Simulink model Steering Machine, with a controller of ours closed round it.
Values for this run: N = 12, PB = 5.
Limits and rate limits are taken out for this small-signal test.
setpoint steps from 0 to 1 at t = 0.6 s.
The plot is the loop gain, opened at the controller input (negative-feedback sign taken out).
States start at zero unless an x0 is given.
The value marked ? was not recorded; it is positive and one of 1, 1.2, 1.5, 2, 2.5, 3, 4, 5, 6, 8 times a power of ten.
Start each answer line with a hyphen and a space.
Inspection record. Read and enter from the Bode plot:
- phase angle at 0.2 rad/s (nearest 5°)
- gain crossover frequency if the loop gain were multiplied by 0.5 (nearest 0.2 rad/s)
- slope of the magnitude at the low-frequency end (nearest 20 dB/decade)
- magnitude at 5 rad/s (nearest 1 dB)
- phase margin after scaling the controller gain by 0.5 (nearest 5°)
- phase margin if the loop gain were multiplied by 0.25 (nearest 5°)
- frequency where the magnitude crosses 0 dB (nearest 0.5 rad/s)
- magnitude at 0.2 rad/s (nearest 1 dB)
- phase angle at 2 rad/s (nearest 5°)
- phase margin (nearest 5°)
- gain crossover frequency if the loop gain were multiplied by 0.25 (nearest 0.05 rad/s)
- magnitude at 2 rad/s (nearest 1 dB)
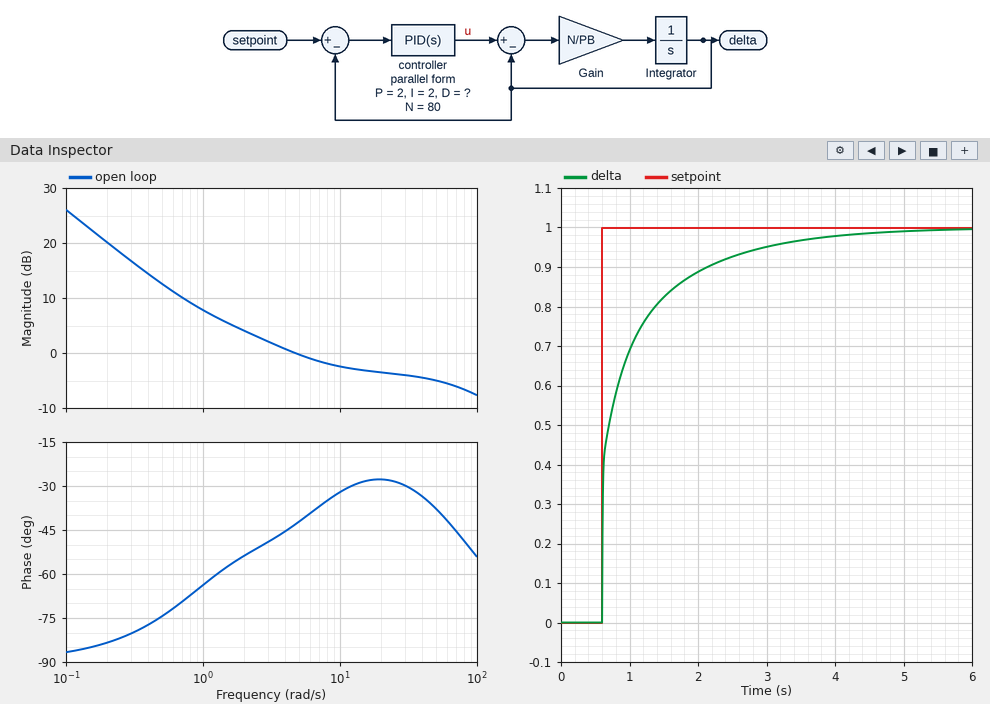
- -85°
- 1.4 rad/s
- -20 dB/decade
- 0 dB
- 120°
- 105°
- 4.5 rad/s
- 20 dB
- -55°
- 135°
- 0.55 rad/s
- 4 dB
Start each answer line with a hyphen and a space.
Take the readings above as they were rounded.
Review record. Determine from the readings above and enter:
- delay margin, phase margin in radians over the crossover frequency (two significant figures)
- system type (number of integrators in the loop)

- 0.52 s
- 1
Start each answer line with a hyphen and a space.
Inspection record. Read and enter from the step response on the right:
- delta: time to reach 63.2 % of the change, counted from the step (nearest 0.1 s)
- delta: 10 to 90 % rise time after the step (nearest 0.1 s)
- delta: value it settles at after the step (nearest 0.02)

- 0.3 s
- 1.5 s
- 1.00
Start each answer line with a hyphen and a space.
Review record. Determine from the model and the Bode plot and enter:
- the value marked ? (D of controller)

- 0.25
